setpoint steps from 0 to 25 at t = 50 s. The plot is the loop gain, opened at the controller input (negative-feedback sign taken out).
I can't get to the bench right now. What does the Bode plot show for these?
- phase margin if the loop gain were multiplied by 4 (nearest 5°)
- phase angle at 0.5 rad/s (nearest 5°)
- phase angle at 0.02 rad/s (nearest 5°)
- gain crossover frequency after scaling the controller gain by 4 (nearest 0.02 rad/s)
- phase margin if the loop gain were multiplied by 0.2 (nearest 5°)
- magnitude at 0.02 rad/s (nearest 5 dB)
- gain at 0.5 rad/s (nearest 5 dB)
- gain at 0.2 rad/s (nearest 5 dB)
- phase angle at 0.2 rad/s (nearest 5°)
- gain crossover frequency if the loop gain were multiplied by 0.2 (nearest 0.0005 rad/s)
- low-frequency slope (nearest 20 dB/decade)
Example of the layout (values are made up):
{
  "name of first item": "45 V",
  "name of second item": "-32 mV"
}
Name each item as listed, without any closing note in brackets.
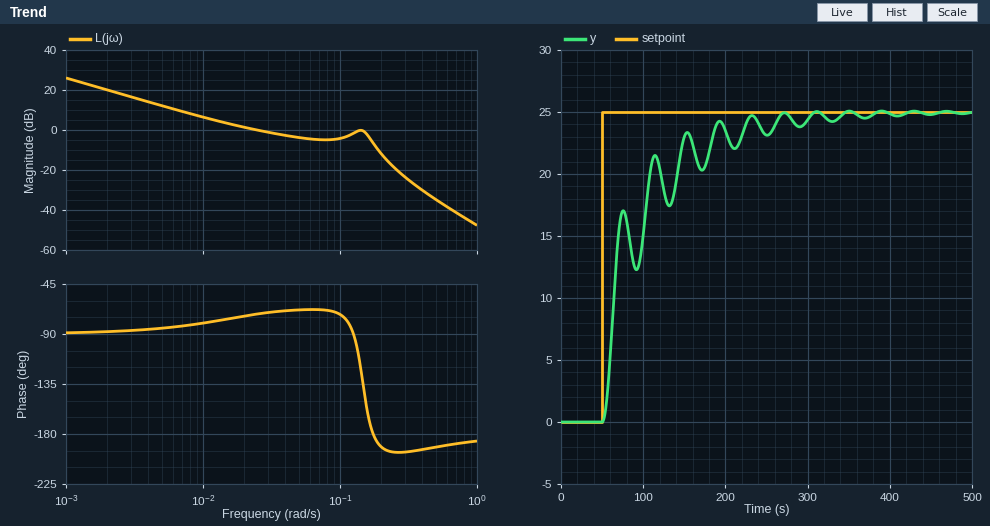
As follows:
{
  "phase margin if the loop gain were multiplied by 4": "-10°",
  "phase angle at 0.5 rad/s": "-190°",
  "phase angle at 0.02 rad/s": "-75°",
  "gain crossover frequency after scaling the controller gain by 4": "0.20 rad/s",
  "phase margin if the loop gain were multiplied by 0.2": "95°",
  "magnitude at 0.02 rad/s": "0 dB",
  "gain at 0.5 rad/s": "-35 dB",
  "gain at 0.2 rad/s": "-10 dB",
  "phase angle at 0.2 rad/s": "-190°",
  "gain crossover frequency if the loop gain were multiplied by 0.2": "0.0040 rad/s",
  "low-frequency slope": "-20 dB/decade"
}
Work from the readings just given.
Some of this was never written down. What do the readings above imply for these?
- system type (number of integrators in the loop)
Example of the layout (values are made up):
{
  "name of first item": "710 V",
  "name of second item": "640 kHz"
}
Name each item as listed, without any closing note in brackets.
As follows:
{
  "system type": "1"
}
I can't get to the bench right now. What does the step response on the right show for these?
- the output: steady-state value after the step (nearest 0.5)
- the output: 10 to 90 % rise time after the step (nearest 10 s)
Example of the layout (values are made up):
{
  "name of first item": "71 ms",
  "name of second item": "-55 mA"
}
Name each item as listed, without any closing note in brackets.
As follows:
{
  "the output: steady-state value after the step": "25.0",
  "the output: 10 to 90 % rise time after the step": "90 s"
}
